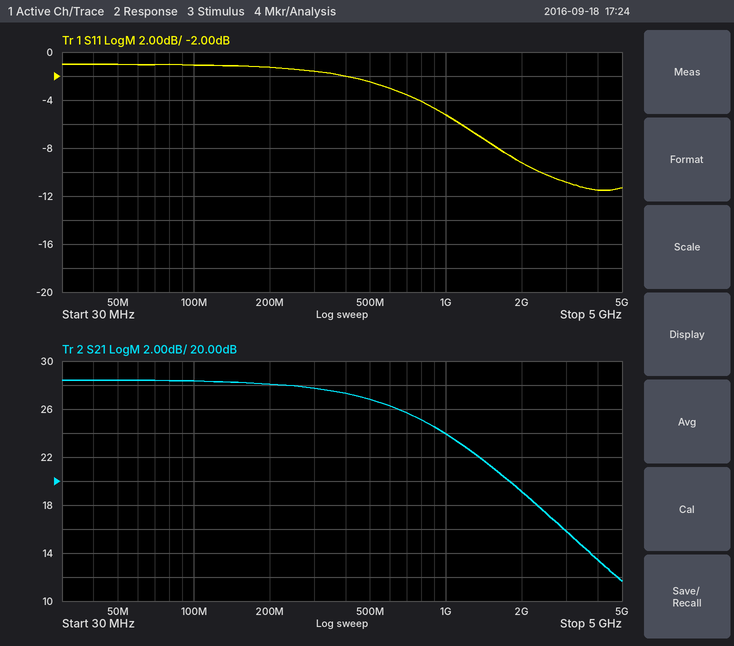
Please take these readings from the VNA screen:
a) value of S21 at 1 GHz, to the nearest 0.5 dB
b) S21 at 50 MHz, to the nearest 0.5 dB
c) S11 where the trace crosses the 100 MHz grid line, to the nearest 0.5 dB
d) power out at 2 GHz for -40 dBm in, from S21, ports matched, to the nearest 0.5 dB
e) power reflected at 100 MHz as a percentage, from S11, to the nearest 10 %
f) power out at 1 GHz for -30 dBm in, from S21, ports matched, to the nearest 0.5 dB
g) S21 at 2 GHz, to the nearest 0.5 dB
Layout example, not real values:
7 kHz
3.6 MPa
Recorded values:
24.0 dB
28.5 dB
-1.0 dB
-21.0 dBm
80 %
-6.0 dBm
19.0 dB
